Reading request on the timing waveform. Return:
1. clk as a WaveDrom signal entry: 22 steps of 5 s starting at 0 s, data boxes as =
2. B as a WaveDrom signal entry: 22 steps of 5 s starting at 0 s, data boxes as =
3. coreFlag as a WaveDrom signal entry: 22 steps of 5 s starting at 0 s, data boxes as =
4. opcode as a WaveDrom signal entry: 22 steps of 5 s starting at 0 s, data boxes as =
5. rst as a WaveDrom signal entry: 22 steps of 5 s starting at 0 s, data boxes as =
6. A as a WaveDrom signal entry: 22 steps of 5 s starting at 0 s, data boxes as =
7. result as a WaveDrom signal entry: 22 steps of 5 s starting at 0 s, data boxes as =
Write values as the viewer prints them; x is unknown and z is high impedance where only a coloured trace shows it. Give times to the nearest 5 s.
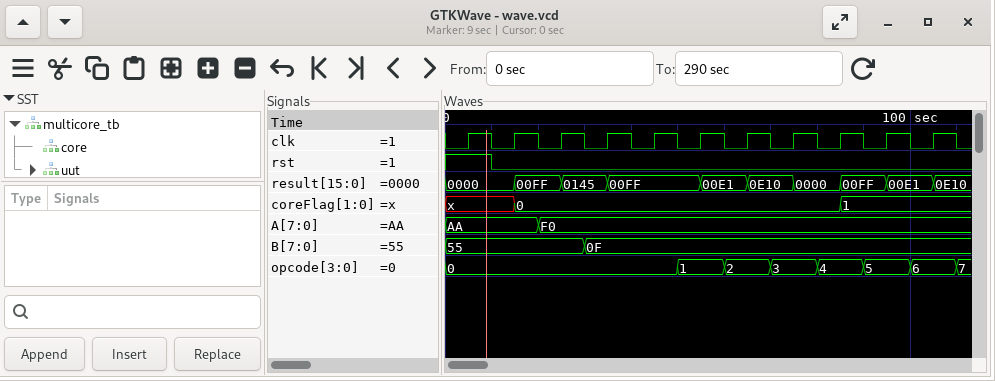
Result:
{name: 'clk', wave: '0101010101010101010101'}
{name: 'B', wave: '=.....=...............', data: '55 0F'}
{name: 'coreFlag', wave: 'x..=.............=....', data: '0 1'}
{name: 'opcode', wave: '=.........=.=.=.=.=.=.', data: '0 1 2 3 4 5 6'}
{name: 'rst', wave: '1.0...................'}
{name: 'A', wave: '=...=.................', data: 'AA F0'}
{name: 'result', wave: '=..=.=.=...=.=.=.=.=.=', data: '0000 00FF 0145 00FF 00E1 0E10 0000 00FF 00E1 0E10'}
